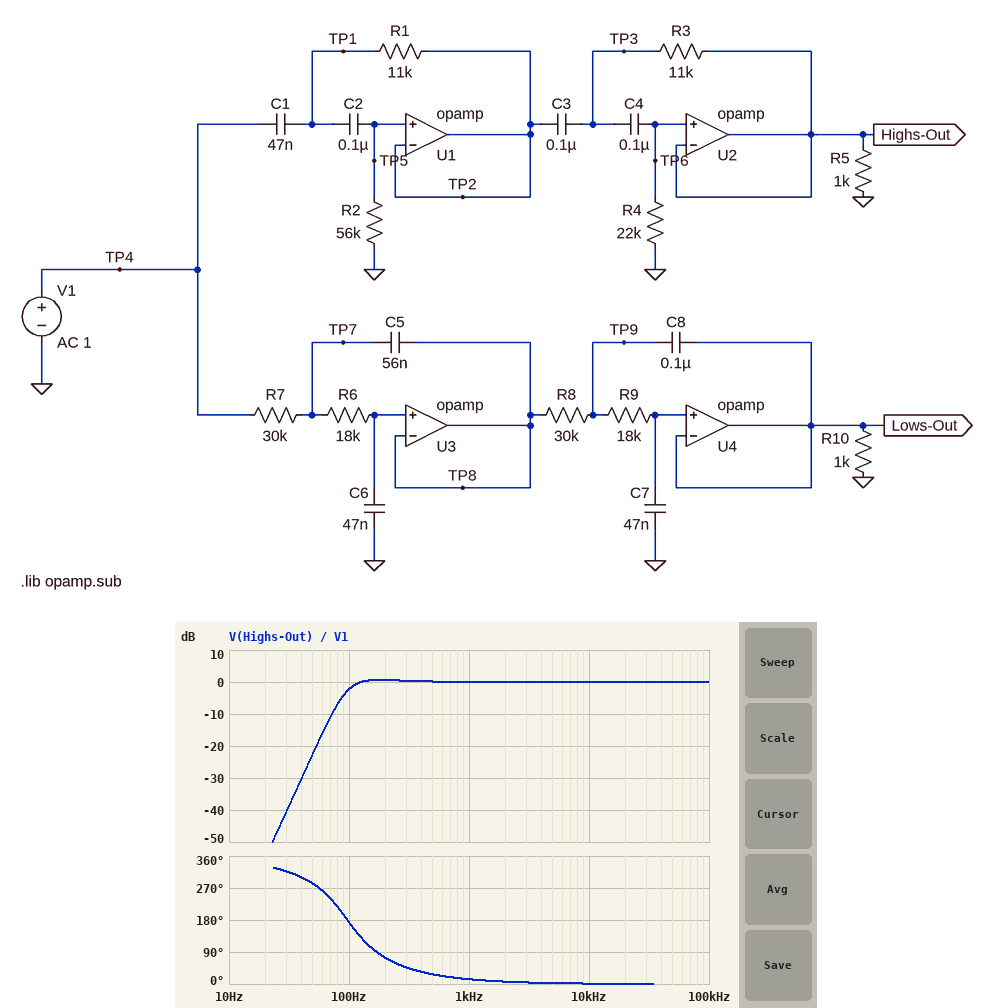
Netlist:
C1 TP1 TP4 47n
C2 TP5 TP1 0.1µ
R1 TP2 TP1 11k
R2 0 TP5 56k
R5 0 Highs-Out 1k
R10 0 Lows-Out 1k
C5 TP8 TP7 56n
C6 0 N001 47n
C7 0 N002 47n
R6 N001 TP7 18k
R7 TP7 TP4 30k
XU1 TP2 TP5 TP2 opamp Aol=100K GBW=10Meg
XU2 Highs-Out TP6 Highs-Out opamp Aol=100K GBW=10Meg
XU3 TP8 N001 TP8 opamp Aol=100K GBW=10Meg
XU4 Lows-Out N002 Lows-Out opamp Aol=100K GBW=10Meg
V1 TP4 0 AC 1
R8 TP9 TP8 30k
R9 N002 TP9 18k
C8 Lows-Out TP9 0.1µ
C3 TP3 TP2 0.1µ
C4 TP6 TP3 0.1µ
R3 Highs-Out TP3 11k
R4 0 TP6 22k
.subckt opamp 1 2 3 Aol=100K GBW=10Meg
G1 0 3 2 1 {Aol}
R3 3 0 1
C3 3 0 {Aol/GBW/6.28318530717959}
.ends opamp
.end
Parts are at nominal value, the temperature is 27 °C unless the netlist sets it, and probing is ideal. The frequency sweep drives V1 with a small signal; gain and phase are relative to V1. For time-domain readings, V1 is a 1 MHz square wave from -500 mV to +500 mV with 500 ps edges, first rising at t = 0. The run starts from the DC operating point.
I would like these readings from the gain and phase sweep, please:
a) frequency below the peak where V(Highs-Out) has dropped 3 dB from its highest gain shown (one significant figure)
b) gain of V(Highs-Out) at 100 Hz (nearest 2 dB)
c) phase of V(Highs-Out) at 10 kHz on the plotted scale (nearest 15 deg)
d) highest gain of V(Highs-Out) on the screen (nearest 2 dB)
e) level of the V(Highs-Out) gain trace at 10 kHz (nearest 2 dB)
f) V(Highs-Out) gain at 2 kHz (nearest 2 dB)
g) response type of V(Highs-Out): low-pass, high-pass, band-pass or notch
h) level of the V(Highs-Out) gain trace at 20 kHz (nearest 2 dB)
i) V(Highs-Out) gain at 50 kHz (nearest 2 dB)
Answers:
100 Hz
-2 dB
0 deg
0 dB
0 dB
0 dB
high-pass
0 dB
0 dB
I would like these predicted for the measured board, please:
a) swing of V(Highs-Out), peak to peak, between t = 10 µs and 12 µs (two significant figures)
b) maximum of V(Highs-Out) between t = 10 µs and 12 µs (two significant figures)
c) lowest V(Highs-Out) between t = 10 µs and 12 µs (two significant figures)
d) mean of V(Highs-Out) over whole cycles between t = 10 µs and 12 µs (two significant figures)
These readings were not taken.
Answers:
1.0 V
990 mV
-8.8 mV
490 mV
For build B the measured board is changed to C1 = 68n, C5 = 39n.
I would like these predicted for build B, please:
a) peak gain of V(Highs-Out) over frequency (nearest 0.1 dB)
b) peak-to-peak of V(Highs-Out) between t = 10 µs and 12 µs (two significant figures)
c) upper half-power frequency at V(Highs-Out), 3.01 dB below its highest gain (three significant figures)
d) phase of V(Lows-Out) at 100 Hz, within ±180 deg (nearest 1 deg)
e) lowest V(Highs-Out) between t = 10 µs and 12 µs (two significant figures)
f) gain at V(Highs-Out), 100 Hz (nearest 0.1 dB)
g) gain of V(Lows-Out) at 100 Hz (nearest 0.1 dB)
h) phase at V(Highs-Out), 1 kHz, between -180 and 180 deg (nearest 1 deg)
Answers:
0.5 dB
1.0 V
5.84 MHz
-157 deg
-8.1 mV
-1.3 dB
-6.8 dB
12 deg
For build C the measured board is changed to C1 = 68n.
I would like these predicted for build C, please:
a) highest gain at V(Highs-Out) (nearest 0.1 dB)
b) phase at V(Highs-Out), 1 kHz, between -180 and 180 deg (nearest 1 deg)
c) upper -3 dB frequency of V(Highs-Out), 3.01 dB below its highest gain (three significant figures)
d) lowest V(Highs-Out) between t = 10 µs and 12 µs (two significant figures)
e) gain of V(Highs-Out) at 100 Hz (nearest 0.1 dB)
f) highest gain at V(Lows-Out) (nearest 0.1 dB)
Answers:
0.5 dB
12 deg
5.84 MHz
-8.1 mV
-1.3 dB
0 dB
